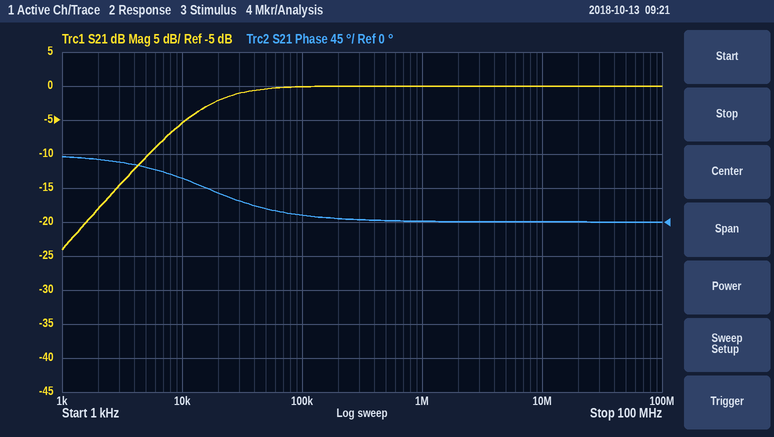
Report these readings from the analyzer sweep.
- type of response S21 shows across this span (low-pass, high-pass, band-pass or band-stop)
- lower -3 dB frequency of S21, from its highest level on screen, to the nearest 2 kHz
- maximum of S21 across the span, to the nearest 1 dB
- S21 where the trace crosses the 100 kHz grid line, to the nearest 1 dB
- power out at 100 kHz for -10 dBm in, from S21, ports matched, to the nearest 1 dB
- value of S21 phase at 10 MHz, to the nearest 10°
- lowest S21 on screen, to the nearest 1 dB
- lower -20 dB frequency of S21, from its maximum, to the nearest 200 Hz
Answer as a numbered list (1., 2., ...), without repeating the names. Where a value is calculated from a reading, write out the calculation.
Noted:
1. high-pass
2. 16 kHz
3. 0 dB
4. 0 dB
5. -10 dBm + (0 dB) = -10 dBm
6. 0°
7. -24 dB
8. 1.6 kHz
